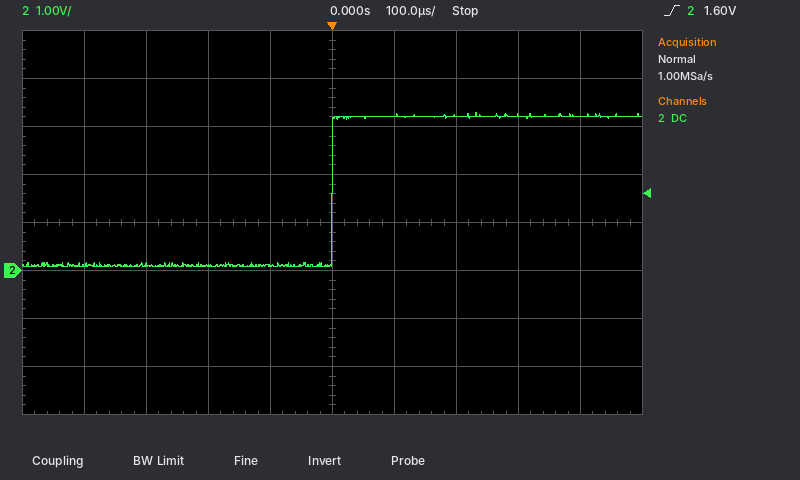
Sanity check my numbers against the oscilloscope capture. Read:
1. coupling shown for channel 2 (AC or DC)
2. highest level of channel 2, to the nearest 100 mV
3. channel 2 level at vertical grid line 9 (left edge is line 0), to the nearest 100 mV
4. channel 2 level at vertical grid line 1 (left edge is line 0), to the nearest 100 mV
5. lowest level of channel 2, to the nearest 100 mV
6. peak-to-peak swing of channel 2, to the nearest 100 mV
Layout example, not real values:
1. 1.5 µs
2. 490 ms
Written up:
1. DC
2. 3.3 V
3. 3.2 V
4. 100 mV
5. 100 mV
6. 3.2 V
